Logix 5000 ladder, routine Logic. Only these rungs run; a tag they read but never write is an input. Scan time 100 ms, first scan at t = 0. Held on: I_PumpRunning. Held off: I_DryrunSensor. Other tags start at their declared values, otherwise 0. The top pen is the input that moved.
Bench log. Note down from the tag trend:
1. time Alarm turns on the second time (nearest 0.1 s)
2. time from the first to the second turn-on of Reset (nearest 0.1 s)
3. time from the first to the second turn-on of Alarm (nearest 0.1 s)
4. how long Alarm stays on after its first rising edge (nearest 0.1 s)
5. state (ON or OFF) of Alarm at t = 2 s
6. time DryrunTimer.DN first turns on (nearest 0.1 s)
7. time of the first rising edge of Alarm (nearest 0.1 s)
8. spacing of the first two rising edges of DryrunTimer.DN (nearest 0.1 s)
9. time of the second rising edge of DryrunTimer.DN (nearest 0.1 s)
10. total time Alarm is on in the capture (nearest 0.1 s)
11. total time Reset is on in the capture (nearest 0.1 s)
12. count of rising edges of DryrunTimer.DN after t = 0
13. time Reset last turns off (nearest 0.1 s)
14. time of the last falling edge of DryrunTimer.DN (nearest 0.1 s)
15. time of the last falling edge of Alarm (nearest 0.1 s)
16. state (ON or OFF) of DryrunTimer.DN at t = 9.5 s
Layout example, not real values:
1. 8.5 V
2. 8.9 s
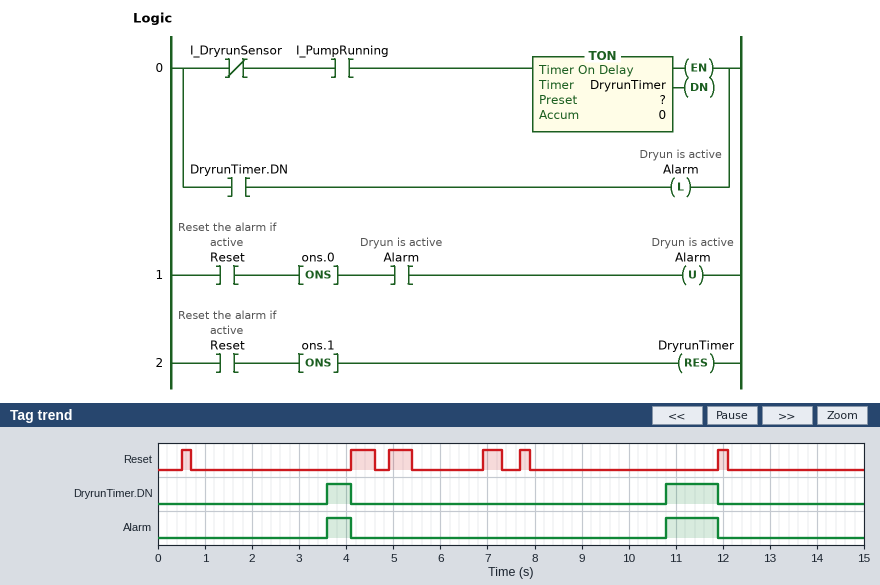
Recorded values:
1. 10.8 s
2. 3.6 s
3. 7.2 s
4. 0.5 s
5. OFF
6. 3.6 s
7. 3.6 s
8. 7.2 s
9. 10.8 s
10. 1.6 s
11. 2.0 s
12. 2
13. 12.1 s
14. 11.9 s
15. 11.9 s
16. OFF
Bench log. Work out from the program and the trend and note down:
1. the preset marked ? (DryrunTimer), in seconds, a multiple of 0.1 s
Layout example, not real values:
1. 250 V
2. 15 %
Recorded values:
1. 3.0 s
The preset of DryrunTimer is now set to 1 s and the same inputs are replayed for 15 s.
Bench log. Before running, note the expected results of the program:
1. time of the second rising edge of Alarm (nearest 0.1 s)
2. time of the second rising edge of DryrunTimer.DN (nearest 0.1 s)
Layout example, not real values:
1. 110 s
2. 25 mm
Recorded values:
1. 6.0 s
2. 6.0 s
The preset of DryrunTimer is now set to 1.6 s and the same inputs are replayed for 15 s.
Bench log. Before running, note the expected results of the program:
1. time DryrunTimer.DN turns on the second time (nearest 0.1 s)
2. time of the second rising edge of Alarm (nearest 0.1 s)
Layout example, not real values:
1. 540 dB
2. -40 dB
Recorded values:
1. 6.6 s
2. 6.6 s
